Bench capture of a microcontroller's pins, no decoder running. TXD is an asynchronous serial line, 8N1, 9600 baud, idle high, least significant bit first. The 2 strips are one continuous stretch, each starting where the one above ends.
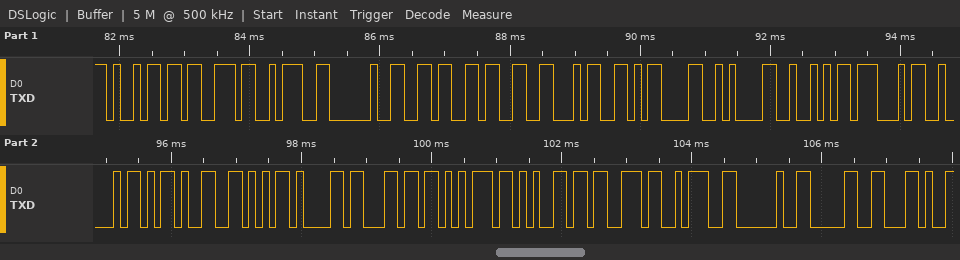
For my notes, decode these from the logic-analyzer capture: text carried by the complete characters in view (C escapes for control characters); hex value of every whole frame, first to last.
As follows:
"is: 634\r\nRGB-Values: 0,"
69 73 3A 20 36 33 34 0D 0A 52 47 42 2D 56 61 6C 75 65 73 3A 20 30 2C
